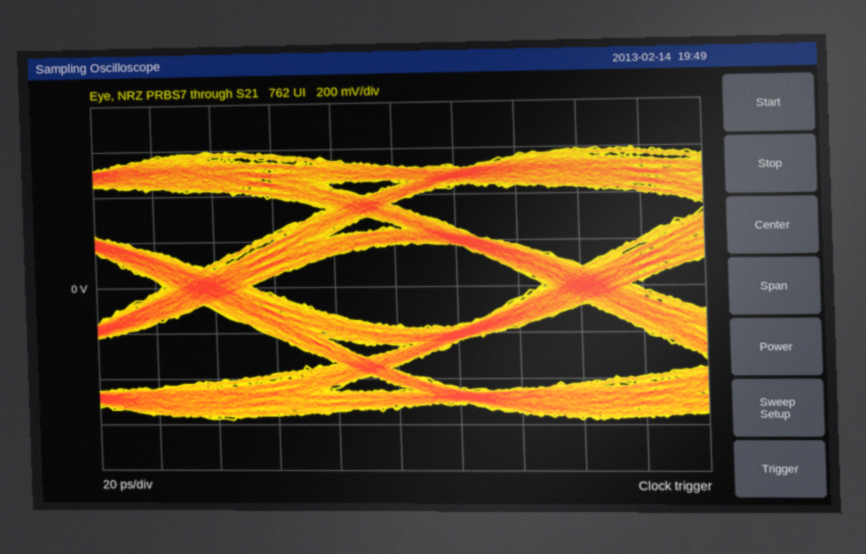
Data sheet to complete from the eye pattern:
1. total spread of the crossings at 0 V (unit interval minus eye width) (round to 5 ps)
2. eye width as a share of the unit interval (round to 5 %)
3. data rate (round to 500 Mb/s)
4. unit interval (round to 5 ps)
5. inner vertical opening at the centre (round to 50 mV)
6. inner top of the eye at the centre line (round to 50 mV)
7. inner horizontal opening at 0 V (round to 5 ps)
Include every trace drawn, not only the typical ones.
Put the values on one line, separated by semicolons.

30 ps; 75 %; 8.0 Gb/s; 125 ps; 350 mV; 200 mV; 95 ps
